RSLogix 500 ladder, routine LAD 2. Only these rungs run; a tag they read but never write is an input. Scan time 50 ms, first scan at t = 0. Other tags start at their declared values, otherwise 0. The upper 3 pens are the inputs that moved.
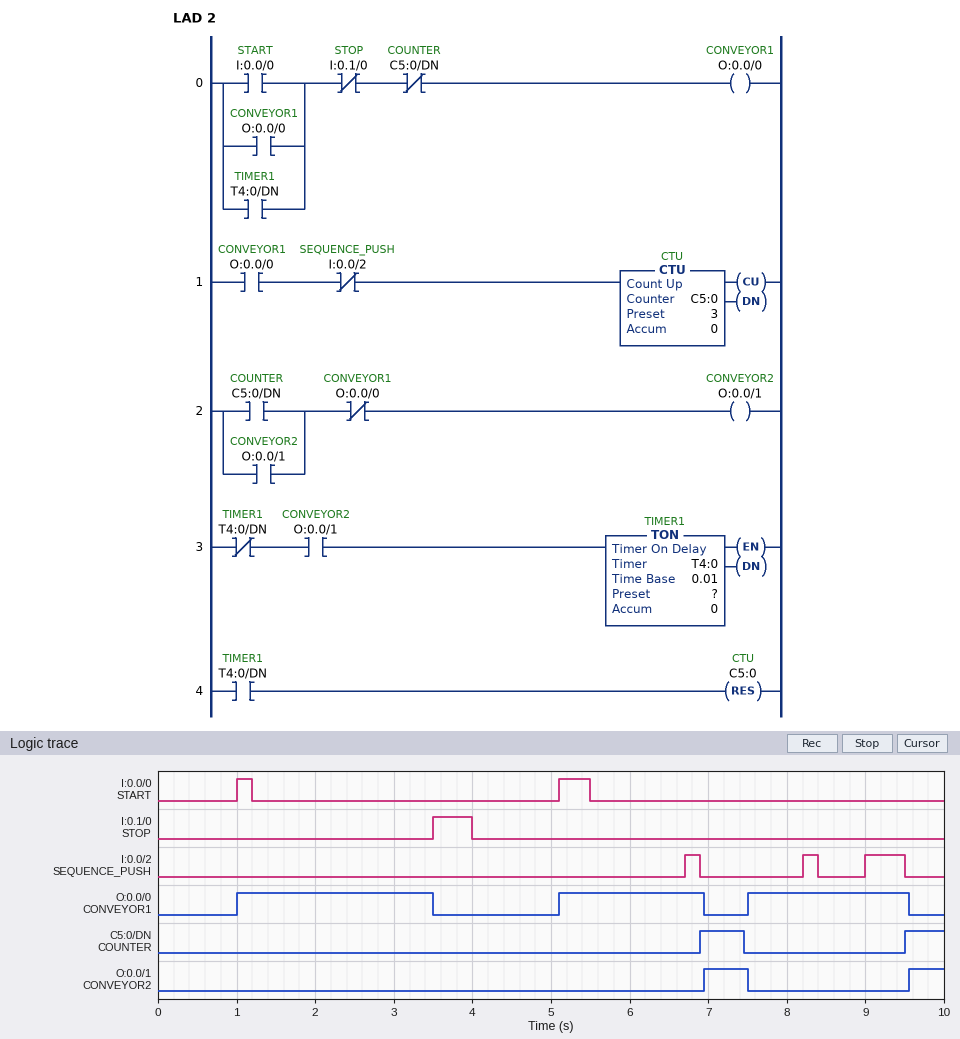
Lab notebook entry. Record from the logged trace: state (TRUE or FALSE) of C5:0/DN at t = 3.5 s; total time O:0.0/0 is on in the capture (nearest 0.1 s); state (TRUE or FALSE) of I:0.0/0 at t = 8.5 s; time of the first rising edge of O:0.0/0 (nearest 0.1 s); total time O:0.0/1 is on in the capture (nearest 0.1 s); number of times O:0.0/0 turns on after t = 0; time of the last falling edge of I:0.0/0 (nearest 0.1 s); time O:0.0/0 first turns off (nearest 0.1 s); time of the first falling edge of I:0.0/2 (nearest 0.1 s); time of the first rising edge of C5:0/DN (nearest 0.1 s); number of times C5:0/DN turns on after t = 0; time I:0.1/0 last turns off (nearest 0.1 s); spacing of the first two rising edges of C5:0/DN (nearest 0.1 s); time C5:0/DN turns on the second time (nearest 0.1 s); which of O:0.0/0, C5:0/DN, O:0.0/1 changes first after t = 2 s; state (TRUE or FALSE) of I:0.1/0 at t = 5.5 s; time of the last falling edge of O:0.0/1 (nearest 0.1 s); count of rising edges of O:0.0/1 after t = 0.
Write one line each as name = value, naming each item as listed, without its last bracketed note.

state (TRUE or FALSE) of C5:0/DN at t = 3.5 s = FALSE
total time O:0.0/0 is on in the capture = 6.4 s
state (TRUE or FALSE) of I:0.0/0 at t = 8.5 s = FALSE
time of the first rising edge of O:0.0/0 = 1.0 s
total time O:0.0/1 is on in the capture = 1.0 s
number of times O:0.0/0 turns on after t = 0 = 3
time of the last falling edge of I:0.0/0 = 5.5 s
time O:0.0/0 first turns off = 3.5 s
time of the first falling edge of I:0.0/2 = 6.9 s
time of the first rising edge of C5:0/DN = 6.9 s
number of times C5:0/DN turns on after t = 0 = 2
time I:0.1/0 last turns off = 4.0 s
spacing of the first two rising edges of C5:0/DN = 2.6 s
time C5:0/DN turns on the second time = 9.5 s
which of O:0.0/0, C5:0/DN, O:0.0/1 changes first after t = 2 s = O:0.0/0
state (TRUE or FALSE) of I:0.1/0 at t = 5.5 s = FALSE
time of the last falling edge of O:0.0/1 = 7.5 s
count of rising edges of O:0.0/1 after t = 0 = 2
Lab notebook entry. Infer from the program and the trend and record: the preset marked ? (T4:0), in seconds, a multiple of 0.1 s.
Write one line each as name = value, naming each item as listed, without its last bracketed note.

the preset marked ? (T4:0), in seconds, a multiple of 0.1 s = 0.5 s
